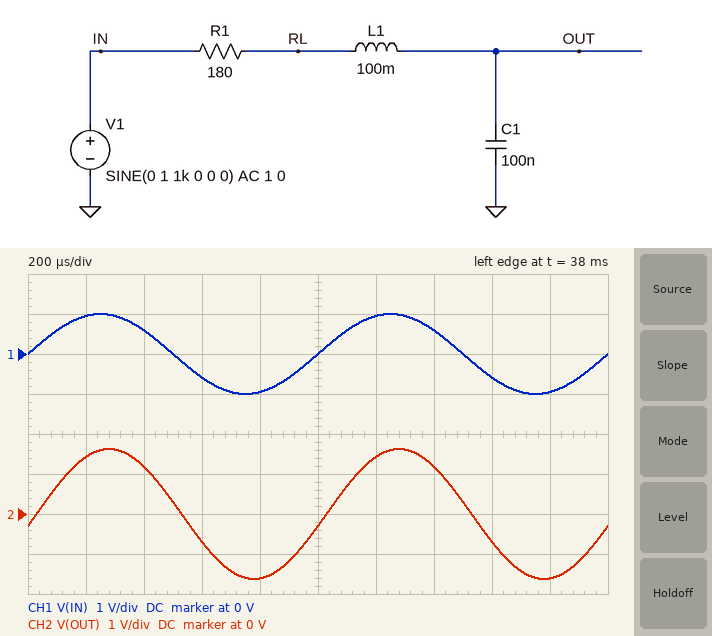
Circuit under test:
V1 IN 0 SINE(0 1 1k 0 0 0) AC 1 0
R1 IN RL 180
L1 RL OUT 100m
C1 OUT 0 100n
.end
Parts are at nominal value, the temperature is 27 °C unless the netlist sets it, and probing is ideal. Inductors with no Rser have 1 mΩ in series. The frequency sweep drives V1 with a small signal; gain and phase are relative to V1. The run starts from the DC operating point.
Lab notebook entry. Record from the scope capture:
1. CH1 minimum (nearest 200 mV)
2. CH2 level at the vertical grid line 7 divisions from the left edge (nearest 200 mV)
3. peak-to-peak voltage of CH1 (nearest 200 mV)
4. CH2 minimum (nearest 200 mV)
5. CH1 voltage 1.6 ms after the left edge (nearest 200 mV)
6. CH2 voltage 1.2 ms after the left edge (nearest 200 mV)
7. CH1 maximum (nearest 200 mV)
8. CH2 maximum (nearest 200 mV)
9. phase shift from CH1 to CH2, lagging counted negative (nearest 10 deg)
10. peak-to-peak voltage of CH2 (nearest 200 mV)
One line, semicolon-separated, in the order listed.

-1.0 V; 1.2 V; 2.0 V; -1.6 V; -600 mV; 1.4 V; 1.0 V; 1.6 V; -10 deg; 3.2 V
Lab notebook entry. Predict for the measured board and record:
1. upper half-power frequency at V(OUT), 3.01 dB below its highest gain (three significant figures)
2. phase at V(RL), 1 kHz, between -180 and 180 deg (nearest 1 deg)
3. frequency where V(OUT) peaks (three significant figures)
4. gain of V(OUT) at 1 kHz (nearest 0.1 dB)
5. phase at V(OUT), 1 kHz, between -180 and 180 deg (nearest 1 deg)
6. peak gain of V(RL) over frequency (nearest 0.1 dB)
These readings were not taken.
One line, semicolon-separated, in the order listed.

1.72 kHz; -11 deg; 1.58 kHz; 4.2 dB; -11 deg; 0 dB
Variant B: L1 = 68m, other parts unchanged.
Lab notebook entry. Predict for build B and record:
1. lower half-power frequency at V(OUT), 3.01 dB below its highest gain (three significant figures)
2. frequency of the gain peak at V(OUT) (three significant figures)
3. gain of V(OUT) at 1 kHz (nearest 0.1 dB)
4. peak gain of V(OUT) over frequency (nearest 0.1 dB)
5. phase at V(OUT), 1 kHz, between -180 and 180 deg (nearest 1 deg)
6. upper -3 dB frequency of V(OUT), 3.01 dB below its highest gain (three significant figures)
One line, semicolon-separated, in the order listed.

1.68 kHz; 1.91 kHz; 2.6 dB; 13.3 dB; -9 deg; 2.11 kHz
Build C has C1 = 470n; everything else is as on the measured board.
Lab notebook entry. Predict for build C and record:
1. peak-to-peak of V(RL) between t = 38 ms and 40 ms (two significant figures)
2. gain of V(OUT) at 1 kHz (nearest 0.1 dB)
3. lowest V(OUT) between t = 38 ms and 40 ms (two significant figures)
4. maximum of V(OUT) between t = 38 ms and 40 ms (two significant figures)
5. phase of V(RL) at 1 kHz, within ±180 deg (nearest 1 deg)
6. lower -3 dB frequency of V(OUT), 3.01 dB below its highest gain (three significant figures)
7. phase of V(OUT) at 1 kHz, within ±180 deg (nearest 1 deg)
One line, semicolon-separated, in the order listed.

1.7 V; -0.1 dB; -990 mV; 990 mV; 32 deg; 540 Hz; -148 deg
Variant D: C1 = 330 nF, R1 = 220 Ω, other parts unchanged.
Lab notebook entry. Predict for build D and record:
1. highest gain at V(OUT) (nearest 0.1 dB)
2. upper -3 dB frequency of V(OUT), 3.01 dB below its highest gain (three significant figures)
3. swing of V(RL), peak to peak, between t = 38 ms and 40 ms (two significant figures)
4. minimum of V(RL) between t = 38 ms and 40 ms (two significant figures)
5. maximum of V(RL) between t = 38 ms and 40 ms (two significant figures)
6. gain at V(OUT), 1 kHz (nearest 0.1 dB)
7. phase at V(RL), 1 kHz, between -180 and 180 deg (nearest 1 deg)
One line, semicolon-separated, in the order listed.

8.1 dB; 1.00 kHz; 1.1 V; -550 mV; 550 mV; 5.2 dB; 56 deg
